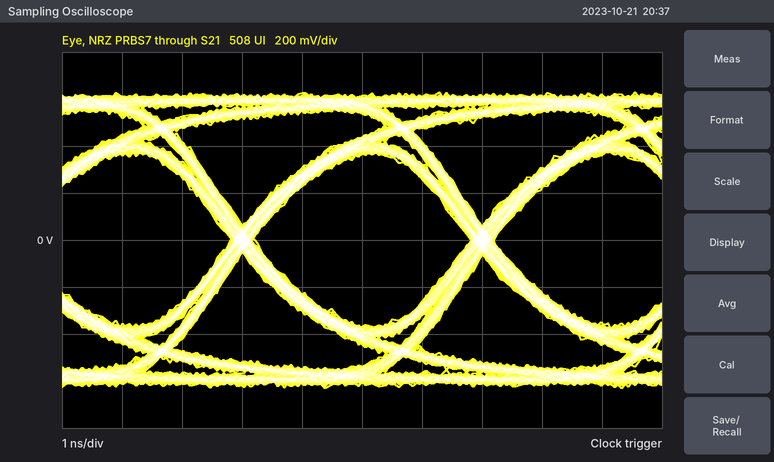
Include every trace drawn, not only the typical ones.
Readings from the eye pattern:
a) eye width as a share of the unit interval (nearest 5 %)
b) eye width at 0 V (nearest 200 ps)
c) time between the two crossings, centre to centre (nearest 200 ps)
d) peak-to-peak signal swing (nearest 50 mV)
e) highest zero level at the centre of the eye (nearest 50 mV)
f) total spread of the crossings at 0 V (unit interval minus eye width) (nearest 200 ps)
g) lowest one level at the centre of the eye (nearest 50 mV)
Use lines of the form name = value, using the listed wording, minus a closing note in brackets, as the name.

eye width as a share of the unit interval = 90 %
eye width at 0 V = 3.6 ns
time between the two crossings, centre to centre = 4.0 ns
peak-to-peak signal swing = 1.25 V
highest zero level at the centre of the eye = -350 mV
total spread of the crossings at 0 V (unit interval minus eye width) = 400 ps
lowest one level at the centre of the eye = 350 mV
